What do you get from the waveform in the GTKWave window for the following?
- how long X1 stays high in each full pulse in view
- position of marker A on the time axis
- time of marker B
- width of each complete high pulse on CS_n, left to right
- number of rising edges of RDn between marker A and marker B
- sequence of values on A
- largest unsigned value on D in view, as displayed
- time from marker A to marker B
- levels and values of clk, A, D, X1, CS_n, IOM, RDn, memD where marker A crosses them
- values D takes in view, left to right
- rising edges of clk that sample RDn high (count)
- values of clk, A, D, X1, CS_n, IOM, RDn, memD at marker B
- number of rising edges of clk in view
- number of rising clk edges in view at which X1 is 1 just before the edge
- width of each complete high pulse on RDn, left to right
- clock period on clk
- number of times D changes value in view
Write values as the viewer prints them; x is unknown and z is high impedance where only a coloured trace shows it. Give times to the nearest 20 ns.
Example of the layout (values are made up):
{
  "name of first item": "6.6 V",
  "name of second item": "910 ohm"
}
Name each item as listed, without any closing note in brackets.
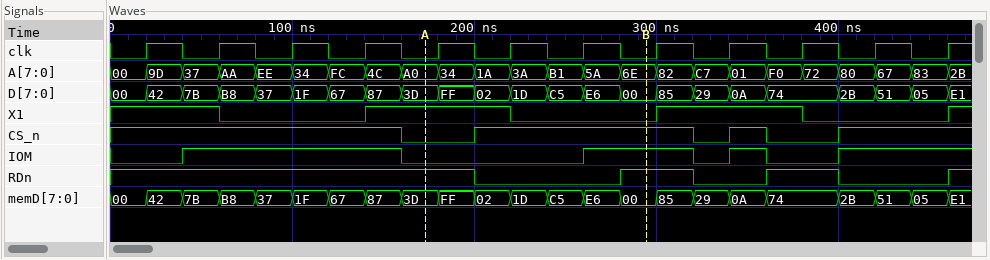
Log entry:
{
  "how long X1 stays high in each full pulse in view": "80 ns, 80 ns",
  "position of marker A on the time axis": "180 ns",
  "time of marker B": "300 ns",
  "width of each complete high pulse on CS_n, left to right": "120 ns, 20 ns",
  "number of rising edges of RDn between marker A and marker B": "1",
  "sequence of values on A": "00, 9D, 37, AA, EE, 34, FC, 4C, A0, 34, 1A, 3A, B1, 5A, 6E, 82, C7, 01, F0, 72, 80, 67, 83, 2B",
  "largest unsigned value on D in view, as displayed": "FF",
  "time from marker A to marker B": "120 ns",
  "levels and values of clk, A, D, X1, CS_n, IOM, RDn, memD where marker A crosses them": "clk=0, A=A0, D=3D, X1=1, CS_n=0, IOM=0, RDn=1, memD=3D",
  "values D takes in view, left to right": "00, 42, 7B, B8, 37, 1F, 67, 87, 3D, FF, 02, 1D, C5, E6, 00, 85, 29, 0A, 74, 2B, 51, 05, E1",
  "rising edges of clk that sample RDn high": "7",
  "values of clk, A, D, X1, CS_n, IOM, RDn, memD at marker B": "clk=0, A=6E, D=00, X1=0, CS_n=1, IOM=1, RDn=1, memD=00",
  "number of rising edges of clk in view": "12",
  "number of rising clk edges in view at which X1 is 1 just before the edge": "6",
  "width of each complete high pulse on RDn, left to right": "40 ns, 40 ns",
  "clock period on clk": "40 ns",
  "number of times D changes value in view": "22"
}
